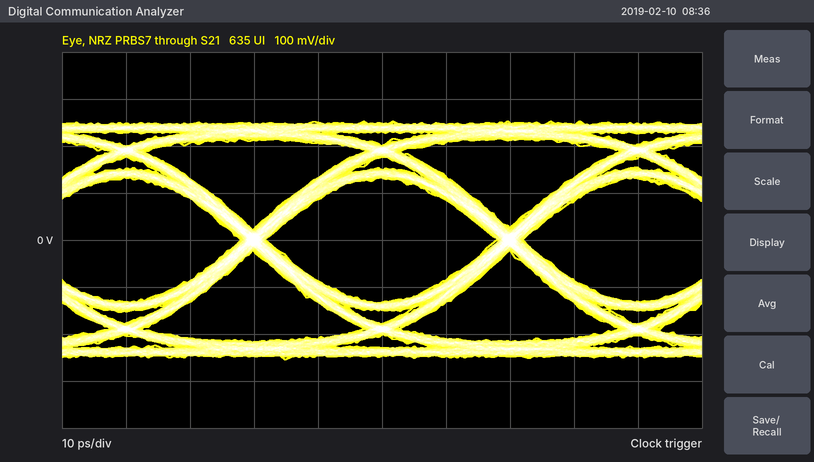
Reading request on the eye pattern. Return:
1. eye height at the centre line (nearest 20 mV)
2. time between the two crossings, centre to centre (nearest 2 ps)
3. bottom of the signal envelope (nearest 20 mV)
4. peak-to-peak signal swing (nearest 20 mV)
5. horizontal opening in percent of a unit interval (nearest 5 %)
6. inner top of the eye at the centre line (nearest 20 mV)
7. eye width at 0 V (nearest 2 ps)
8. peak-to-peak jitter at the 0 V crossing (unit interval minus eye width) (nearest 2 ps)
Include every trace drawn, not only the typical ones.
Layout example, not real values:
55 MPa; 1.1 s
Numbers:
260 mV; 40 ps; -260 mV; 500 mV; 90 %; 140 mV; 36 ps; 4 ps
